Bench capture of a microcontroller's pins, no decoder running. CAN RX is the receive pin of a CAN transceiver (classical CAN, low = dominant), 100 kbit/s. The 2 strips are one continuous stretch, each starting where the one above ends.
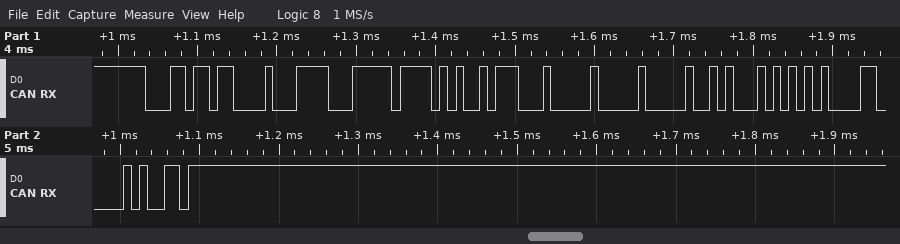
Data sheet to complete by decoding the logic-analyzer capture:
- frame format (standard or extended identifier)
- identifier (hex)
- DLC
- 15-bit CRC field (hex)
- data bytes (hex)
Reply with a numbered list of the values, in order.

1. standard
2. 0x1B6
3. 8
4. 0x0C09
5. F1 FF 52 E2 00 00 A2 AA
